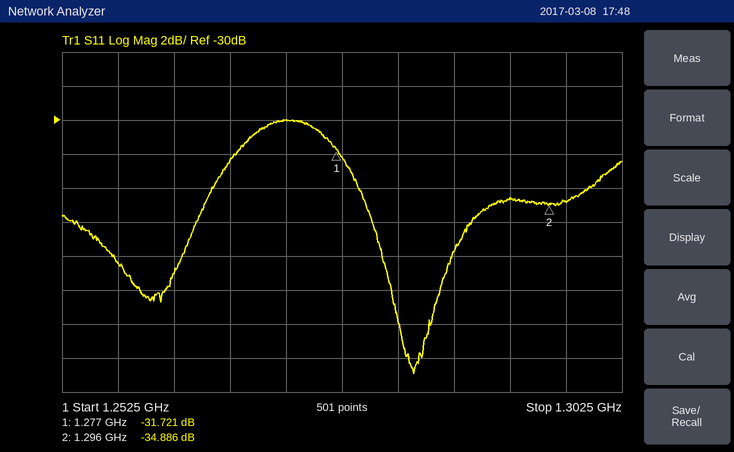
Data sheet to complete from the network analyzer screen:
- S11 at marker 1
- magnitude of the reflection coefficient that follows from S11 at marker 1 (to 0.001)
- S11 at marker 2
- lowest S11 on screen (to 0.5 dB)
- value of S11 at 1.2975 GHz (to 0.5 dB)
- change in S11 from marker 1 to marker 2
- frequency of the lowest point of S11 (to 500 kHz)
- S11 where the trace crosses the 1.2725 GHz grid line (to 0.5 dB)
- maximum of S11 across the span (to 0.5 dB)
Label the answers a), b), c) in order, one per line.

a) -31.721 dB
b) 0.026
c) -34.886 dB
d) -45.0 dB
e) -35.0 dB
f) -3.165 dB
g) 1.2840 GHz
h) -30.0 dB
i) -30.0 dB
